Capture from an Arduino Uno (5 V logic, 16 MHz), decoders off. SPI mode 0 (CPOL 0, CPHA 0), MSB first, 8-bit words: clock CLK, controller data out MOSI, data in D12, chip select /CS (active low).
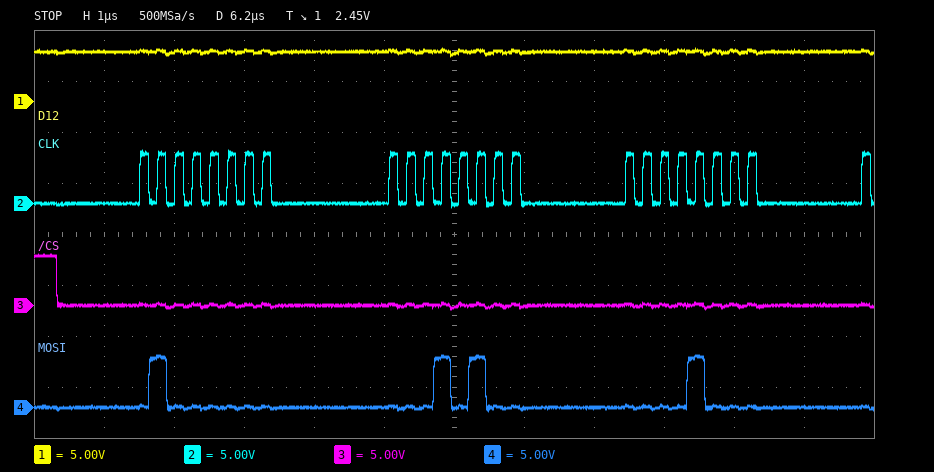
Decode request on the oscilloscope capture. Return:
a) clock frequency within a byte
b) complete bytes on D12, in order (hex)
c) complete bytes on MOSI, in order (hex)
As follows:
4 MHz
FF FF FF
40 14 08
